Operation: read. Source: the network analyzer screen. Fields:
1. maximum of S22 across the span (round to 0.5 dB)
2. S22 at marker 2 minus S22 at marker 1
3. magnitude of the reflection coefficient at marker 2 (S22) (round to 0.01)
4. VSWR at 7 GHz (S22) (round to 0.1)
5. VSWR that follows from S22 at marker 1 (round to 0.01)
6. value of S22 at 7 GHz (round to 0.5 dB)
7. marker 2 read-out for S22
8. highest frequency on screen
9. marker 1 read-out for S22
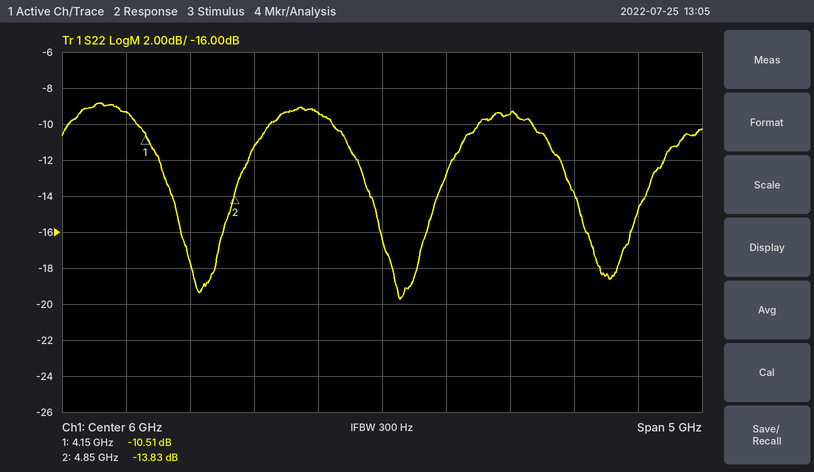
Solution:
-9.0 dB
-3.32 dB
0.20
2.0
1.85
-9.5 dB
-13.83 dB
8.5 GHz
-10.51 dB
